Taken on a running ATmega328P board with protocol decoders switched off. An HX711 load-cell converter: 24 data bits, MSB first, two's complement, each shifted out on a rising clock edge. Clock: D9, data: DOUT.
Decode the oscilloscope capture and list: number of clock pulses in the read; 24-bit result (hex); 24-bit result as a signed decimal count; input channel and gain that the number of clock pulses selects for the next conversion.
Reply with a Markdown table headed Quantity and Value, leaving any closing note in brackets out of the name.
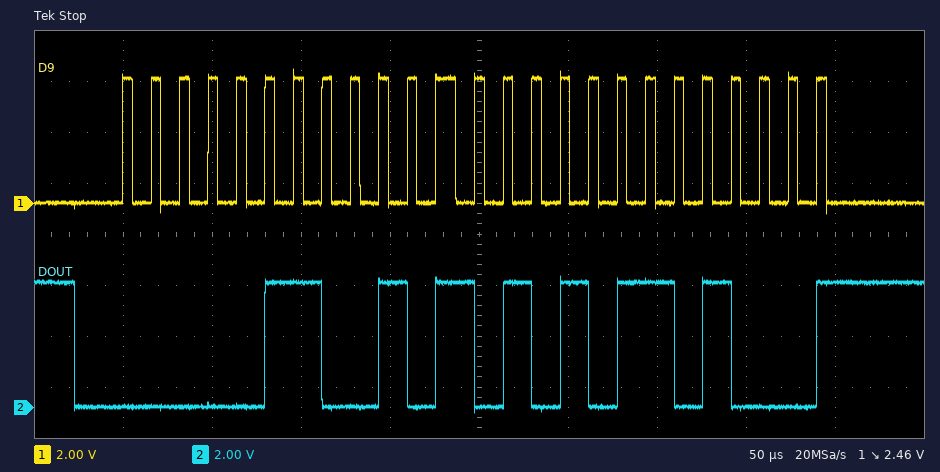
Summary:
| Quantity | Value |
|---|---|
| number of clock pulses in the read | 25 |
| 24-bit result | 0x065568 |
| 24-bit result as a signed decimal count | 415080 |
| input channel and gain that the number of clock pulses selects for the next conversion | channel A, gain 128 |
